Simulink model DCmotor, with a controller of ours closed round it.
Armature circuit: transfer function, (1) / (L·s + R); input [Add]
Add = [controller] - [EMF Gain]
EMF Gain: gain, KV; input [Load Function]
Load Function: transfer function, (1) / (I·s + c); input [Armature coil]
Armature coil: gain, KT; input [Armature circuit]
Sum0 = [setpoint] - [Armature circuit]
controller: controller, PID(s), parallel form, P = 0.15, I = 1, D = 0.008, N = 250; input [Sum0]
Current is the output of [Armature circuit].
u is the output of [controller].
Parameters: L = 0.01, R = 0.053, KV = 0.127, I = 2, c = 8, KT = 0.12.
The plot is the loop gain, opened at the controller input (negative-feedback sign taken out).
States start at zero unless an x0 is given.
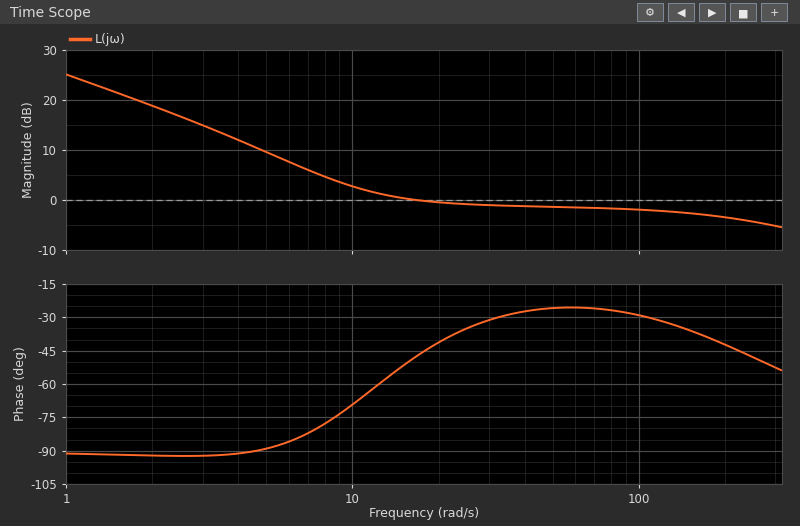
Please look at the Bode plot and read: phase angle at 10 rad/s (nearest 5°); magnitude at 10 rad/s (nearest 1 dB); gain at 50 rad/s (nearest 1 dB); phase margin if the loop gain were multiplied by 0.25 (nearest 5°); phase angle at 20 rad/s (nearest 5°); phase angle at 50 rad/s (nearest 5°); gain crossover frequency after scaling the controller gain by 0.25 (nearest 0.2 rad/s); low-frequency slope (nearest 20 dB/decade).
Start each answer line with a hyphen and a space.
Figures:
- -70°
- 3 dB
- -1 dB
- 90°
- -40°
- -25°
- 4.0 rad/s
- -20 dB/decade
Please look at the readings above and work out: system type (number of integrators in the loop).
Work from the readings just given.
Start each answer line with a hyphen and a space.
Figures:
- 1
